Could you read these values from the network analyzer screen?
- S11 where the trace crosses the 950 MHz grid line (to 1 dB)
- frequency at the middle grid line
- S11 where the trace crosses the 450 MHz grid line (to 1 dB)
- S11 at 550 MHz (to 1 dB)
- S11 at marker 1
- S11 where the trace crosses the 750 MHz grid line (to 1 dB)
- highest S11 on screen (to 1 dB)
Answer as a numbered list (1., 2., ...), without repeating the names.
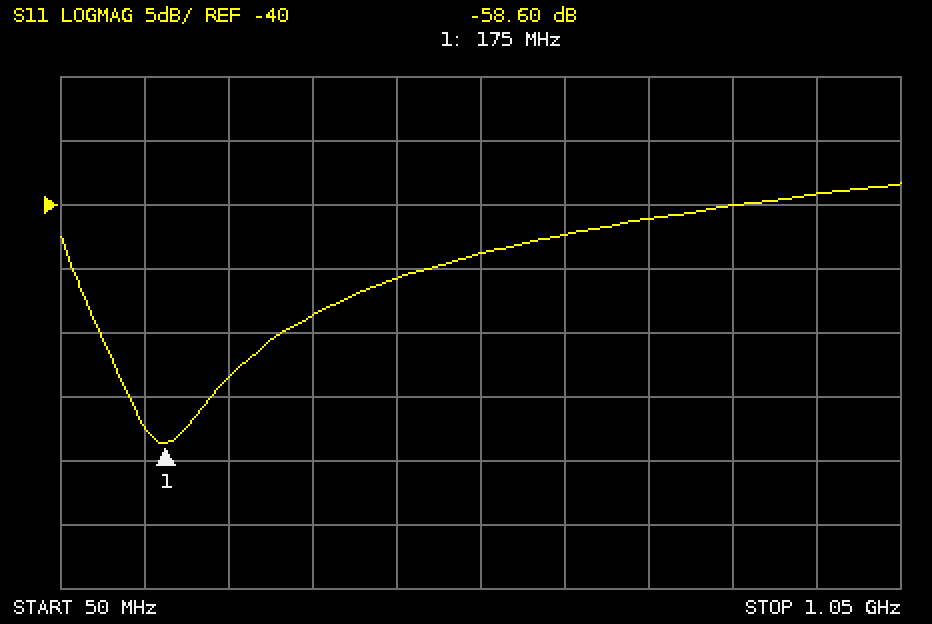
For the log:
1. -39 dB
2. 550 MHz
3. -46 dB
4. -44 dB
5. -58.60 dB
6. -41 dB
7. -38 dB
